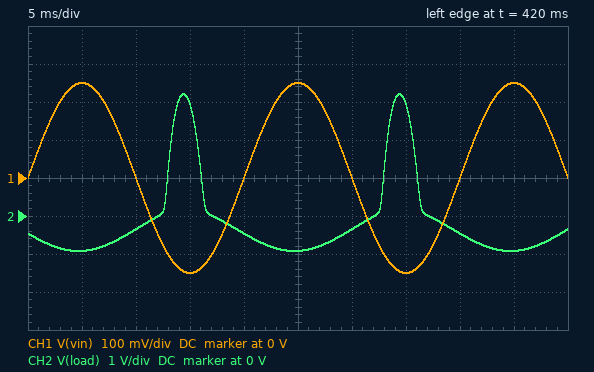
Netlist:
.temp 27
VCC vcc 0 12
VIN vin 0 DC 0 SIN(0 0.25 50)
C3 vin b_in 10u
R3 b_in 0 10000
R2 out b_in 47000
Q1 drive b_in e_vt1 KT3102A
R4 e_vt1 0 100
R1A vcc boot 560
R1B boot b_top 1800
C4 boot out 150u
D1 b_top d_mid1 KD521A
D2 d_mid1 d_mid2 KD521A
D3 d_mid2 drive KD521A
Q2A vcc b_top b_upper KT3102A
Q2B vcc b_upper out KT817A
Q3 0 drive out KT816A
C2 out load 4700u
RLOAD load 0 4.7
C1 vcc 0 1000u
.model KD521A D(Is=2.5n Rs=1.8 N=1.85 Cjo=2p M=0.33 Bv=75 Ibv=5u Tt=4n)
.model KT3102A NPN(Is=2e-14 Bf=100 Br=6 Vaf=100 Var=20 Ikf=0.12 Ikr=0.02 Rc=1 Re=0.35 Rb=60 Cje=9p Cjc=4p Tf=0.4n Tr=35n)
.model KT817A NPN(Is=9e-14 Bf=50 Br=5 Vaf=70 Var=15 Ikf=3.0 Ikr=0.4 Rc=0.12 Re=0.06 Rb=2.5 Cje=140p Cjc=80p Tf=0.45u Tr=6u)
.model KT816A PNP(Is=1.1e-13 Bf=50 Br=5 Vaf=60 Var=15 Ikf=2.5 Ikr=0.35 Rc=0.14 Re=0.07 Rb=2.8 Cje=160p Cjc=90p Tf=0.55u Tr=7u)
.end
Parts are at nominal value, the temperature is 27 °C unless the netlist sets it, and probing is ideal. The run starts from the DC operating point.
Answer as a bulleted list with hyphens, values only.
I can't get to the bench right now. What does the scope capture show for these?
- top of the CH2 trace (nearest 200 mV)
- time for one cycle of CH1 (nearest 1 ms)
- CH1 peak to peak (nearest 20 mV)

- 3.2 V
- 20 ms
- 500 mV
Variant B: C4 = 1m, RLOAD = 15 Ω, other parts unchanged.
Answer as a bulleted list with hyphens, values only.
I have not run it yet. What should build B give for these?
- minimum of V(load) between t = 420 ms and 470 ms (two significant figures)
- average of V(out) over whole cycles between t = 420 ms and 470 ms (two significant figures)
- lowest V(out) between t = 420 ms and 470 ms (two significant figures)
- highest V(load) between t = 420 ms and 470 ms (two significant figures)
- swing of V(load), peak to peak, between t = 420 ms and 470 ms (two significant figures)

- -2.5 V
- 7.1 V
- 4.5 V
- 4.2 V
- 6.7 V
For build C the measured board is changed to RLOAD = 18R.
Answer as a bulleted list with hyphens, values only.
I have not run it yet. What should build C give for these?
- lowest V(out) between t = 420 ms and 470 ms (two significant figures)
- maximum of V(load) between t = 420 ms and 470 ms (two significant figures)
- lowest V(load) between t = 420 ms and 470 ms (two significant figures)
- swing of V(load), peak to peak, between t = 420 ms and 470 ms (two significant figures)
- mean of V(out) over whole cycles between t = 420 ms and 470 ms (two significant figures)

- 4.0 V
- 4.4 V
- -2.9 V
- 7.3 V
- 6.9 V
